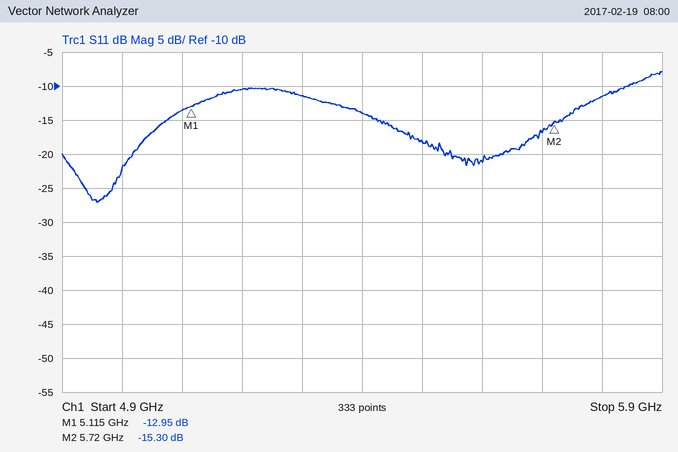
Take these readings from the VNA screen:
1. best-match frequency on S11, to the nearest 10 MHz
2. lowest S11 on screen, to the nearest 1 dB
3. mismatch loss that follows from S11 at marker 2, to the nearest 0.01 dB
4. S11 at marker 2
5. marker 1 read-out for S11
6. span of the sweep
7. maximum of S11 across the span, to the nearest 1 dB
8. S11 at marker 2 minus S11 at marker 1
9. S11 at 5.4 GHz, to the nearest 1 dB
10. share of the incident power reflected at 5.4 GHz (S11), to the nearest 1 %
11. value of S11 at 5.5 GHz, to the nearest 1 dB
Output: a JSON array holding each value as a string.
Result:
["4.96 GHz", "-27 dB", "0.13 dB", "-15.30 dB", "-12.95 dB", "1 GHz", "-8 dB", "-2.35 dB", "-14 dB", "4 %", "-18 dB"]
